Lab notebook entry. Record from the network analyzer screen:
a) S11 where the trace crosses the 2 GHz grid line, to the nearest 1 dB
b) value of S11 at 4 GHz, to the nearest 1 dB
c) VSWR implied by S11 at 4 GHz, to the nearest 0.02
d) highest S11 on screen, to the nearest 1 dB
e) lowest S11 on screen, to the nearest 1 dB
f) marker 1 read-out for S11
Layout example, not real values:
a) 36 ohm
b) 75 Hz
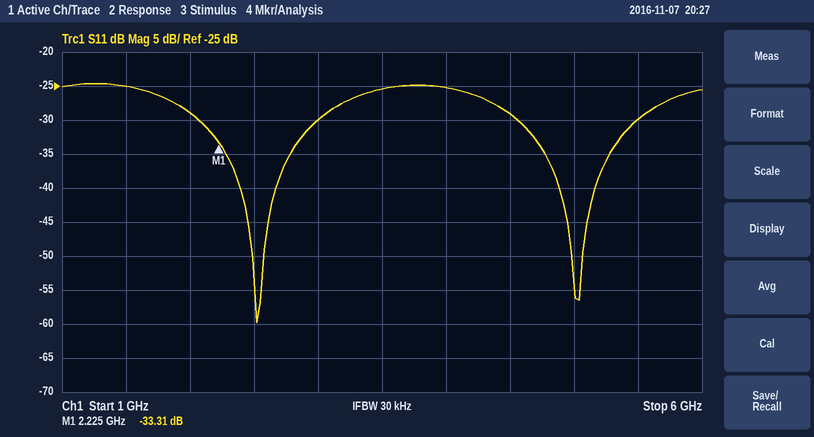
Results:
a) -29 dB
b) -25 dB
c) 1.12
d) -25 dB
e) -60 dB
f) -33.31 dB
